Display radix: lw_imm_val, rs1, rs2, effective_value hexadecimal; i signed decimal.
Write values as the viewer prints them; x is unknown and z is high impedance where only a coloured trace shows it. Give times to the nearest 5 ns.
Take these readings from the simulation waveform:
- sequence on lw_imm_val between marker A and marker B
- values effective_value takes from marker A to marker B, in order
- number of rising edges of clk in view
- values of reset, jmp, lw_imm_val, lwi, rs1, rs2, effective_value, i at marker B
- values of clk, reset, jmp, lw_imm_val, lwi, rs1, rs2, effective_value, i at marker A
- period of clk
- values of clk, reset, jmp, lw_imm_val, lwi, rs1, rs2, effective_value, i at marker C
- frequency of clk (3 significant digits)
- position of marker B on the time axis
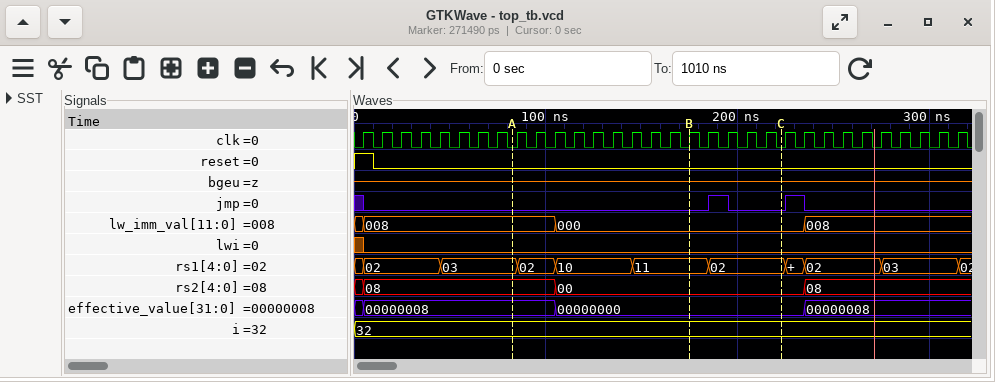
008, 000
00000008, 00000000
32
reset=0, jmp=0, lw_imm_val=000, lwi=0, rs1=11, rs2=00, effective_value=00000000, i=32
clk=0, reset=0, jmp=0, lw_imm_val=008, lwi=0, rs1=03, rs2=08, effective_value=00000008, i=32
10 ns
clk=0, reset=0, jmp=0, lw_imm_val=000, lwi=0, rs1=02, rs2=00, effective_value=00000000, i=32
100 MHz
175 ns
